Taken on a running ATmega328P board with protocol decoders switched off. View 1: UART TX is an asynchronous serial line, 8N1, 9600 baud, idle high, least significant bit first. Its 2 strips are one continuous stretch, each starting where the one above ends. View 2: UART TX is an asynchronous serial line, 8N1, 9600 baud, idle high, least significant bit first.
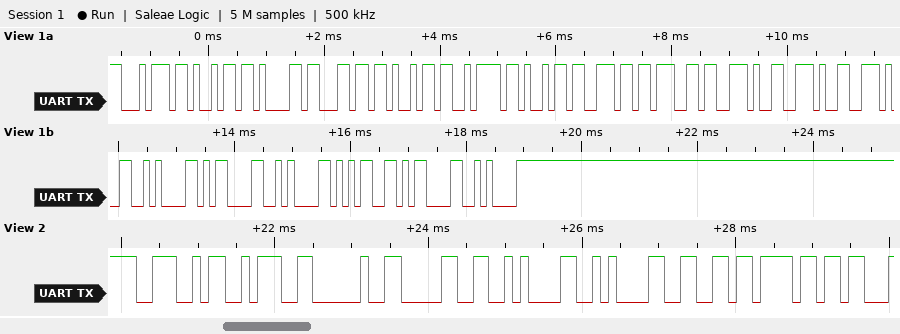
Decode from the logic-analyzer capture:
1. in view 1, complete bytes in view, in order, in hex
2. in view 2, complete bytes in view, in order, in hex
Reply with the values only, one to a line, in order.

74 69 61 6C 69 7A 69 6E 67 2E 2E 2E 0A 0D 0A 35 0D 0A
0x4E 0x3A 0x20 0x30 0x0A 0x0A 0x66 0x6F
